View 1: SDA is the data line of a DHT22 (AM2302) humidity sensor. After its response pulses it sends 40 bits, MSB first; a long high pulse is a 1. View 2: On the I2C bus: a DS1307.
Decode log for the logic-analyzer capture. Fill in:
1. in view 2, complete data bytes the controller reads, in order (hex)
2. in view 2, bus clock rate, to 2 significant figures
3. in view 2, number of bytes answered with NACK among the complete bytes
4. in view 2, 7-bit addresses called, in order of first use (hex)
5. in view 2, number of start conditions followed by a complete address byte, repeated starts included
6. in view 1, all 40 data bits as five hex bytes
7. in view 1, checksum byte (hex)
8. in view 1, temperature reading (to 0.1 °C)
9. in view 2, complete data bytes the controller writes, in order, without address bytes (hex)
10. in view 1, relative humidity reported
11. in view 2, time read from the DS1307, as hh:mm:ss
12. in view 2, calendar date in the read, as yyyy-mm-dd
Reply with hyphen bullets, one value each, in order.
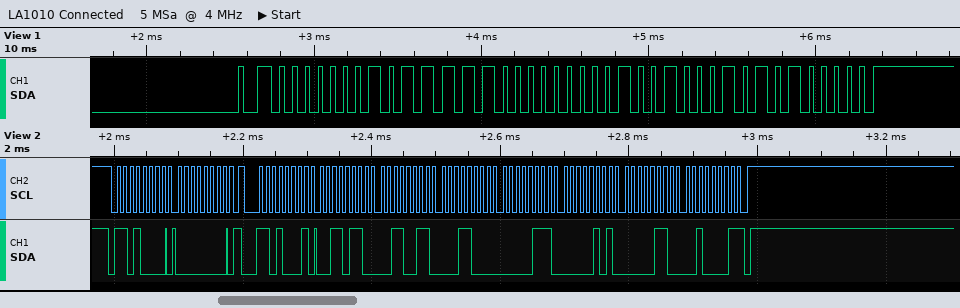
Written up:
- 36 33 18 07 05 06 21
- 100 kHz
- 1
- 0x68
- 2
- 01 7C 01 22 A0
- 0xA0
- 29.0 °C
- 00
- 38.0 %
- 18:33:36
- 2021-06-05
